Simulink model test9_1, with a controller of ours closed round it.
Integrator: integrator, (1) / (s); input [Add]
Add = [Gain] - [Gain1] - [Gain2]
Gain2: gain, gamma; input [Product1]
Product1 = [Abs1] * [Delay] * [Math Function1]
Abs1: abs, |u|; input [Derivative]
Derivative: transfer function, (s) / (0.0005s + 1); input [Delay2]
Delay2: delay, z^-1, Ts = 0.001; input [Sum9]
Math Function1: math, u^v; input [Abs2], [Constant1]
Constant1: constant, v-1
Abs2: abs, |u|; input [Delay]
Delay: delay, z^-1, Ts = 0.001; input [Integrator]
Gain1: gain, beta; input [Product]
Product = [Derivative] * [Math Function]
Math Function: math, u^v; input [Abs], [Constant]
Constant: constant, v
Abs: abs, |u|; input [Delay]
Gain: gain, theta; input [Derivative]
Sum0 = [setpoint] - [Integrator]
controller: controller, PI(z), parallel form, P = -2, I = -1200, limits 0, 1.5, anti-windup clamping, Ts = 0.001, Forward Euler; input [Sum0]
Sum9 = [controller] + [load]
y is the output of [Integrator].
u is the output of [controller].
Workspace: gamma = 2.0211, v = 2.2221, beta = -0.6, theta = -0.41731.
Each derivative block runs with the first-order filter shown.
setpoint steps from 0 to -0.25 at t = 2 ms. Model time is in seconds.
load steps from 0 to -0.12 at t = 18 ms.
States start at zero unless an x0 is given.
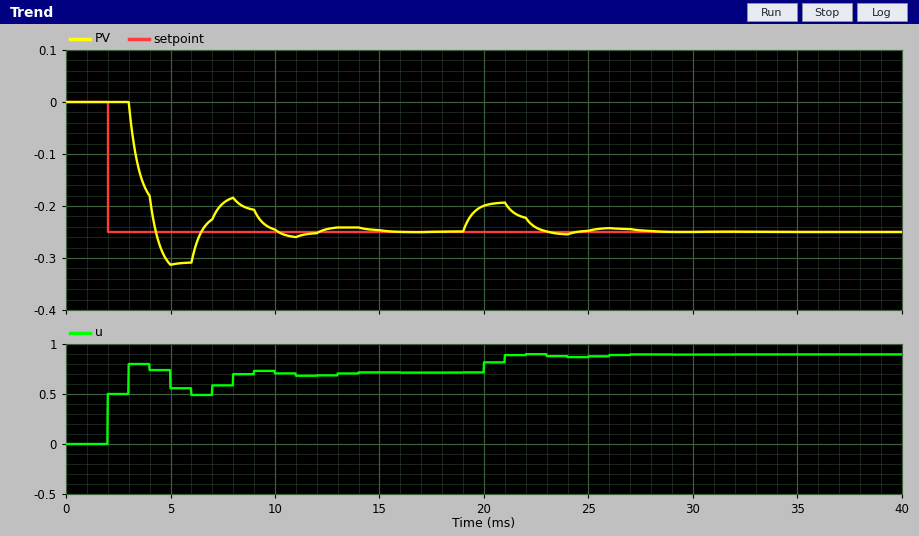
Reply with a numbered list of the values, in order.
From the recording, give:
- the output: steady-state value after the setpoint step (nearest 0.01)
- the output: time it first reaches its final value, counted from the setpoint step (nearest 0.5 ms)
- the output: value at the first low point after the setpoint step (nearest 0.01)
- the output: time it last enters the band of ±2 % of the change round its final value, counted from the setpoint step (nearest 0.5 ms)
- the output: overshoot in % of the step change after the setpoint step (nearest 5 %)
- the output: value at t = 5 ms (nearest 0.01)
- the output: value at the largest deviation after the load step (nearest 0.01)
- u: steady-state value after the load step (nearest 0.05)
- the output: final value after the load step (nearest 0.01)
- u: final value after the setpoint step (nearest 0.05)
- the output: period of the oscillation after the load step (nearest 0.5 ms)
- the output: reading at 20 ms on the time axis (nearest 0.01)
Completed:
1. -0.25
2. 2.5 ms
3. -0.31
4. 12.5 ms
5. 25 %
6. -0.31
7. -0.19
8. 0.90
9. -0.25
10. 0.70
11. 5.0 ms
12. -0.20
